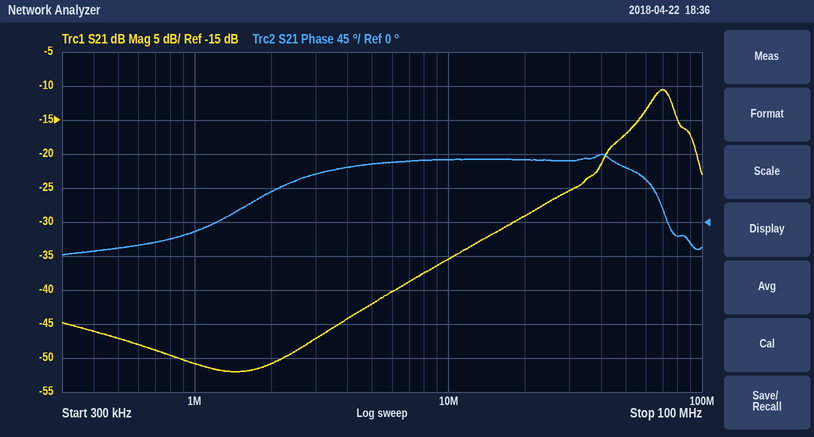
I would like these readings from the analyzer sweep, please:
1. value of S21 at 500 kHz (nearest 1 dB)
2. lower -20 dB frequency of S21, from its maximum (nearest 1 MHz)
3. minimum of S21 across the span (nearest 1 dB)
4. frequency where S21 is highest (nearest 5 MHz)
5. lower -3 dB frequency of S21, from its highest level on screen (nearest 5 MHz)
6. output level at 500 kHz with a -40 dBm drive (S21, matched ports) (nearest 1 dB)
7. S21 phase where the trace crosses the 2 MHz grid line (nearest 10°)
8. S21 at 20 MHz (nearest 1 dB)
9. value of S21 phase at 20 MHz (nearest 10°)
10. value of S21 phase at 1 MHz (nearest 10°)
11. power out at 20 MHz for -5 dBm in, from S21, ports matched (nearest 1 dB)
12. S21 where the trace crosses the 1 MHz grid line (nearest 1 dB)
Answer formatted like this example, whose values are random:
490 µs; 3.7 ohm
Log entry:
-47 dB; 17 MHz; -52 dB; 70 MHz; 60 MHz; -87 dBm; 40°; -29 dB; 80°; -10°; -34 dBm; -51 dB
